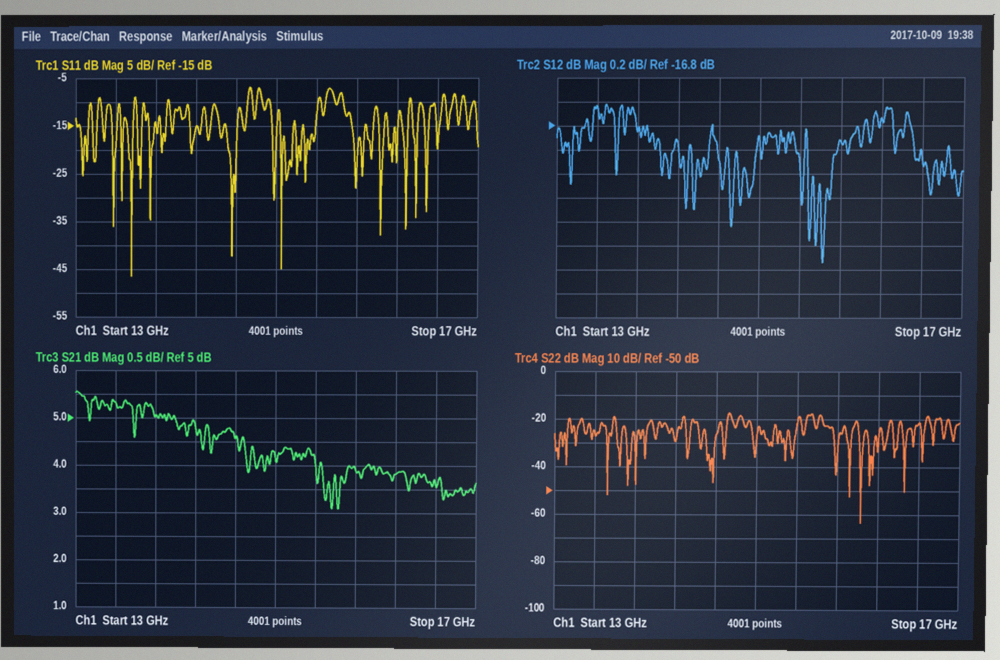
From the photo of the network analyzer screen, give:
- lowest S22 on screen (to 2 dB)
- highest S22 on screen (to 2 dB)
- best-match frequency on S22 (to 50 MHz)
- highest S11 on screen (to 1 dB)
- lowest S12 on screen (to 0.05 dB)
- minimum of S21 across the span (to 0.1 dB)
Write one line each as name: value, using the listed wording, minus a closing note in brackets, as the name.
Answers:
lowest S22 on screen: -64 dB
highest S22 on screen: -18 dB
best-match frequency on S22: 16.05 GHz
highest S11 on screen: -7 dB
lowest S12 on screen: -17.95 dB
minimum of S21 across the span: 3.1 dB
